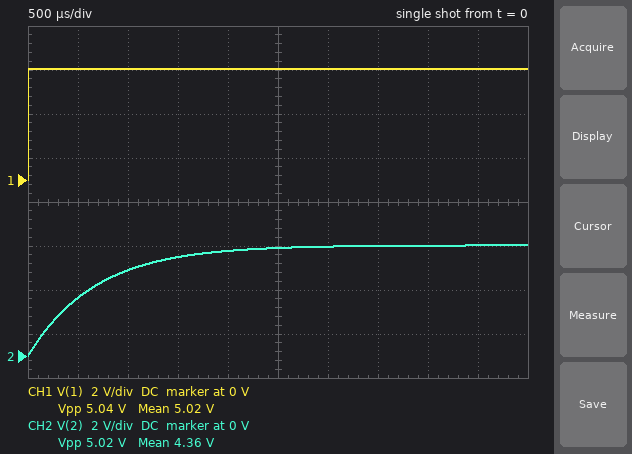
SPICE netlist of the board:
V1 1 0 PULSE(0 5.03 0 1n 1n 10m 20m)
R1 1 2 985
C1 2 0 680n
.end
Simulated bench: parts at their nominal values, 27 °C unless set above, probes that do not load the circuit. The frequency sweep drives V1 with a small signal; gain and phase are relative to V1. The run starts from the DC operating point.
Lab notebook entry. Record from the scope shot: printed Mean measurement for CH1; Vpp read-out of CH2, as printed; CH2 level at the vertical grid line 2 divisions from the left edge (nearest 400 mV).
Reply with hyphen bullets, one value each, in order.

- 5.02 V
- 5.02 V
- 4.0 V
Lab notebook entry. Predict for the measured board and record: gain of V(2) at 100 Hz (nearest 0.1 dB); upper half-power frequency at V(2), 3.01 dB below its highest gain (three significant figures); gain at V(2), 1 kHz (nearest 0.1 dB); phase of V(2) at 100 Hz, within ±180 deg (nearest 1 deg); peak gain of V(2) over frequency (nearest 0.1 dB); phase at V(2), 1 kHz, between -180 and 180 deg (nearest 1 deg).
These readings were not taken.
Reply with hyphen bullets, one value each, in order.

- -0.7 dB
- 238 Hz
- -12.7 dB
- -23 deg
- 0 dB
- -77 deg
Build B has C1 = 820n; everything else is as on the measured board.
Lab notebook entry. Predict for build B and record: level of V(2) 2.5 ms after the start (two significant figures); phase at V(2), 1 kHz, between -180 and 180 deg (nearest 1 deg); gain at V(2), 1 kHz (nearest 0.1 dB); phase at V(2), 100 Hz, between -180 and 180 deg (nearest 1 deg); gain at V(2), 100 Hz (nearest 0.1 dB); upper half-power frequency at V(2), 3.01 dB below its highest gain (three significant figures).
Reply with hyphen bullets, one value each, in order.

- 4.8 V
- -79 deg
- -14.3 dB
- -27 deg
- -1.0 dB
- 197 Hz
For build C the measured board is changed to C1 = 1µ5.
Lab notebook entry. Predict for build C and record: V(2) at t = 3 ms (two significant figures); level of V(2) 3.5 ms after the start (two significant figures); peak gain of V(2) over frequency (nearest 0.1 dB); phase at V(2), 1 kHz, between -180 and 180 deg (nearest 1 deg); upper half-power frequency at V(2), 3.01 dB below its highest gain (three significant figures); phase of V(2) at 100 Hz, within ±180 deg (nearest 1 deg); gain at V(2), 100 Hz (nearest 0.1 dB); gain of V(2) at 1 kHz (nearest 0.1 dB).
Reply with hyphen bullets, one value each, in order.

- 4.4 V
- 4.6 V
- 0 dB
- -84 deg
- 108 Hz
- -43 deg
- -2.7 dB
- -19.4 dB
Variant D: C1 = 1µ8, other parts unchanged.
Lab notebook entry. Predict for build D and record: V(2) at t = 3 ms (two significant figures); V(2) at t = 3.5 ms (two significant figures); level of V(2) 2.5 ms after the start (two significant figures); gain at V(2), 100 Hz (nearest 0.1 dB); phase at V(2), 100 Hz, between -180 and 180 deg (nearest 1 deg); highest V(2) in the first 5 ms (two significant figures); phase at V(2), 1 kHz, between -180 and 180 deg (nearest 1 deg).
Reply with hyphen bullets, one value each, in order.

- 4.1 V
- 4.3 V
- 3.8 V
- -3.5 dB
- -48 deg
- 4.7 V
- -85 deg
